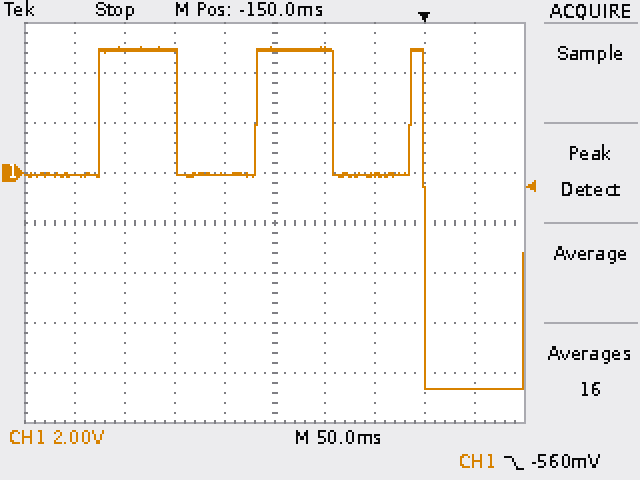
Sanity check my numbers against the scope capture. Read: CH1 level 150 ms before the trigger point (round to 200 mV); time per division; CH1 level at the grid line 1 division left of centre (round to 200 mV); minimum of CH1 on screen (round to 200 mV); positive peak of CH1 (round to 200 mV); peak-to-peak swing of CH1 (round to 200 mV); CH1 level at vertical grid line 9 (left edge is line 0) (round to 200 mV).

5.0 V
50 ms
0.0 V
-8.6 V
5.0 V
13.6 V
-8.6 V
